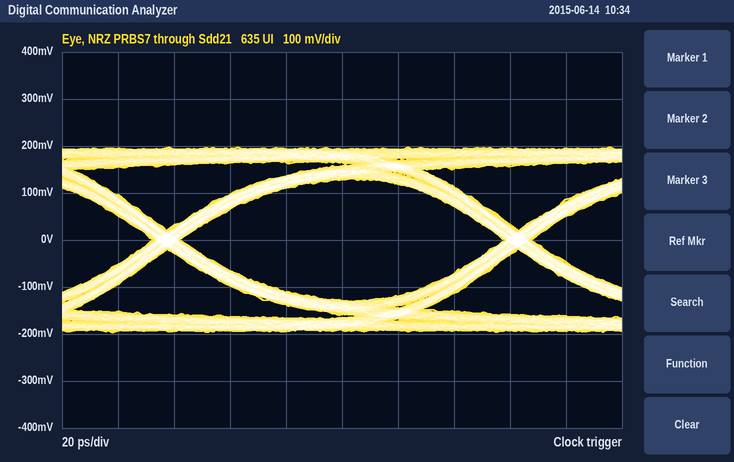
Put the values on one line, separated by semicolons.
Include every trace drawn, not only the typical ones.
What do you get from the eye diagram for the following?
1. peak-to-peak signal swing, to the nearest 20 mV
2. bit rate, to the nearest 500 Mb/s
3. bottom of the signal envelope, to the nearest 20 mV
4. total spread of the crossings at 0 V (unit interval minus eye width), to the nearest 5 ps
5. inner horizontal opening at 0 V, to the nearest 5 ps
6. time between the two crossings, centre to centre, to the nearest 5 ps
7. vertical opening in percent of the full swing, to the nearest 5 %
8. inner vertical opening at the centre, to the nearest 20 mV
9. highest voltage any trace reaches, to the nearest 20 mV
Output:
400 mV; 8.0 Gb/s; -200 mV; 10 ps; 115 ps; 125 ps; 65 %; 260 mV; 200 mV
